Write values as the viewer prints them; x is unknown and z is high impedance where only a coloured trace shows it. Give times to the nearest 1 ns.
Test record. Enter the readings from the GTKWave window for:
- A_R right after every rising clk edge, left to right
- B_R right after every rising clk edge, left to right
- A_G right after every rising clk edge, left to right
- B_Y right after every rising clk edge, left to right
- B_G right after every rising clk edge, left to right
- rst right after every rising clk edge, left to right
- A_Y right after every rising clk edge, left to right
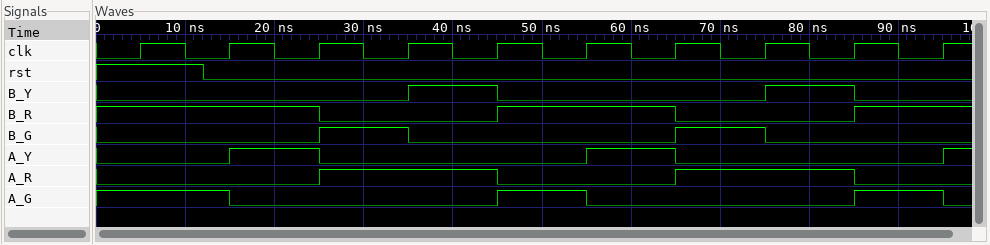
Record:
0 0 1 1 0 0 1 1 0 0
1 1 0 0 1 1 0 0 1 1
1 0 0 0 1 0 0 0 1 0
0 0 0 1 0 0 0 1 0 0
0 0 1 0 0 0 1 0 0 0
1 0 0 0 0 0 0 0 0 0
0 1 0 0 0 1 0 0 0 1
